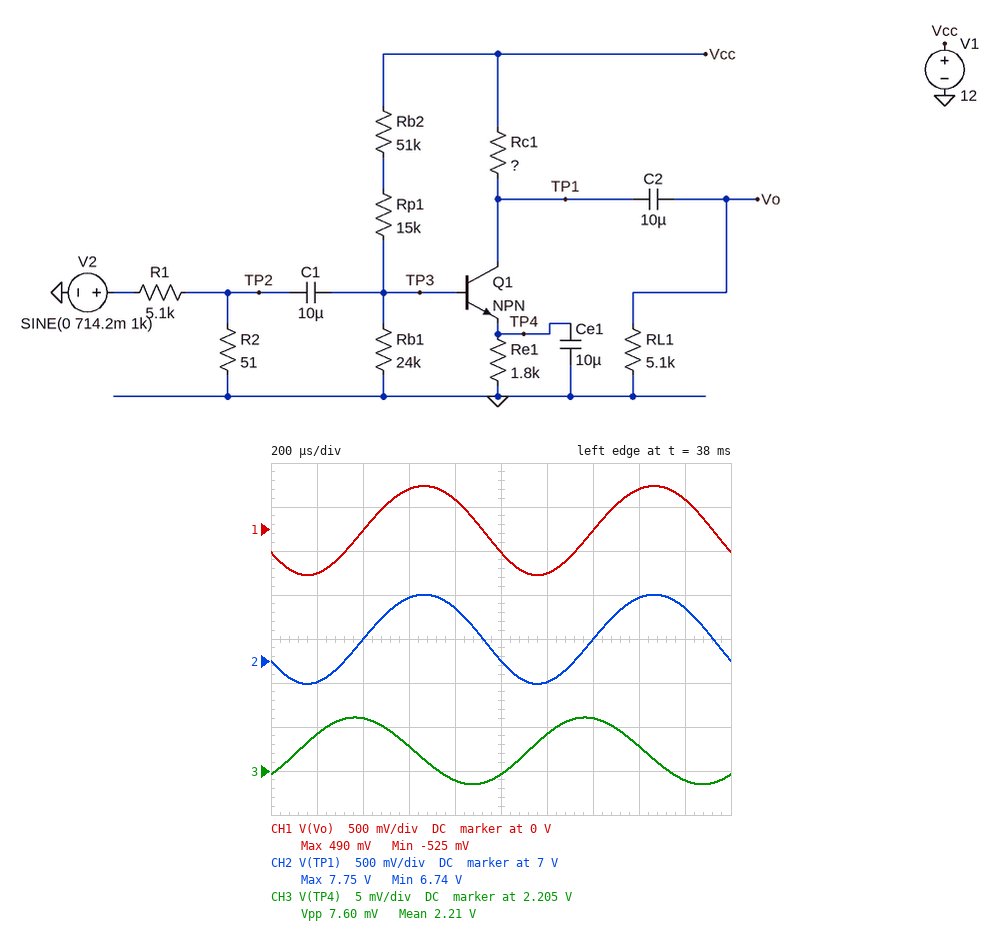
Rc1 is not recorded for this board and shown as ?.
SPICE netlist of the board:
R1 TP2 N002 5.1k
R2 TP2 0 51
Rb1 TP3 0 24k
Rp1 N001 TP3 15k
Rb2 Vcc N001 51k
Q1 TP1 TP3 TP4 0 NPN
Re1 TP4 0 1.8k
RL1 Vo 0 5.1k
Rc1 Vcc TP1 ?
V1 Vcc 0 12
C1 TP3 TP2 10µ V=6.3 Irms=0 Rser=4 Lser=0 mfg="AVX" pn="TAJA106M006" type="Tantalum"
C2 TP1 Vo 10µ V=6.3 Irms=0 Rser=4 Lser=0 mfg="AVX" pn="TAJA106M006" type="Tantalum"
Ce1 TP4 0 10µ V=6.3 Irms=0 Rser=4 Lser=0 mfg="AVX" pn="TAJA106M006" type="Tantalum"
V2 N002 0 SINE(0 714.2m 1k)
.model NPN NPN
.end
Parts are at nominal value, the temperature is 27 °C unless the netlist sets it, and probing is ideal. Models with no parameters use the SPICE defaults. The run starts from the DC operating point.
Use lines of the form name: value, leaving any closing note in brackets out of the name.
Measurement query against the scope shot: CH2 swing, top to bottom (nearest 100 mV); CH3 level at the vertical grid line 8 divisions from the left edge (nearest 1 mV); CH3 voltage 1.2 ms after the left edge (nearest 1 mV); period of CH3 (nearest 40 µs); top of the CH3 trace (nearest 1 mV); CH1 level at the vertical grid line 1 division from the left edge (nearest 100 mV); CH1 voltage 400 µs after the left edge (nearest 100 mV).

CH2 swing, top to bottom: 1.0 V
CH3 level at the vertical grid line 8 divisions from the left edge: 2.208 V
CH3 voltage 1.2 ms after the left edge: 2.209 V
period of CH3: 1.00 ms
top of the CH3 trace: 2.211 V
CH1 level at the vertical grid line 1 division from the left edge: -500 mV
CH1 voltage 400 µs after the left edge: 0 V
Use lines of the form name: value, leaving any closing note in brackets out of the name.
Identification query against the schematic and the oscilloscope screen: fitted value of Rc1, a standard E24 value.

fitted value of Rc1, a standard E24 value: 3.9 kΩ
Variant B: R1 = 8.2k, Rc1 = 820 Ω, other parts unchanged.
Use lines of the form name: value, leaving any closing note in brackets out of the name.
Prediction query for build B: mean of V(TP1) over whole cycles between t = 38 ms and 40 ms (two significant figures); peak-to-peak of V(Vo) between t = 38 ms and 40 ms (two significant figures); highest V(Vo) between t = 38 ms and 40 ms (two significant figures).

mean of V(TP1) over whole cycles between t = 38 ms and 40 ms: 11 V
peak-to-peak of V(Vo) between t = 38 ms and 40 ms: 200 mV
highest V(Vo) between t = 38 ms and 40 ms: 99 mV
